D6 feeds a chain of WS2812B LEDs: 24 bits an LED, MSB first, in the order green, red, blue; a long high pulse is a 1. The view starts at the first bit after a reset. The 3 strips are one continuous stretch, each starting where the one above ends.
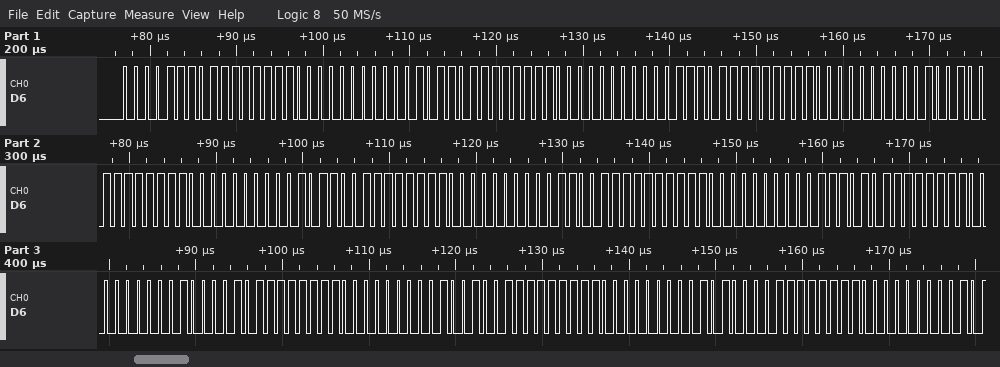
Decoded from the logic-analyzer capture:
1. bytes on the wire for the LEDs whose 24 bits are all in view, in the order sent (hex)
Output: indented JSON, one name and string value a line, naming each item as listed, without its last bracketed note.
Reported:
{
  "bytes on the wire for the LEDs whose 24 bits are all in view, in the order sent": "0E FF 00 16 FF 00 1D FF 00 24 FF 00 2C FF 00 33 FF 00 3A FF 00 42 FF 00 49 FF 00 50 FF 00"
}
